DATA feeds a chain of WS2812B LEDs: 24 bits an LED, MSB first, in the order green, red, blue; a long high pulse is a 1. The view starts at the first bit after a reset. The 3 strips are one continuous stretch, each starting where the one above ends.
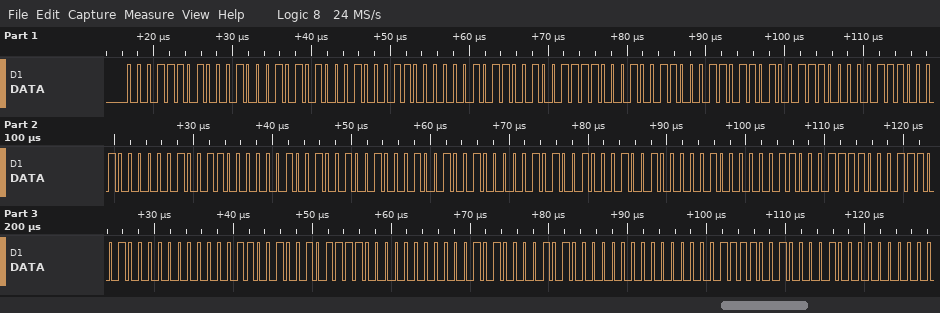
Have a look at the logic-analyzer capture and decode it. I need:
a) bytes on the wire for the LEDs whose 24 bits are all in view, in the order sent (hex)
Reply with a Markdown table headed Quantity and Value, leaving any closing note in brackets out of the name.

| Quantity | Value |
|---|---|
| bytes on the wire for the LEDs whose 24 bits are all in view, in the order sent | 1D 11 51 18 16 4F 13 1B 4E 0E 20 4C 09 24 49 05 22 41 03 1E 39 00 19 2F 00 14 28 00 0F 21 |
